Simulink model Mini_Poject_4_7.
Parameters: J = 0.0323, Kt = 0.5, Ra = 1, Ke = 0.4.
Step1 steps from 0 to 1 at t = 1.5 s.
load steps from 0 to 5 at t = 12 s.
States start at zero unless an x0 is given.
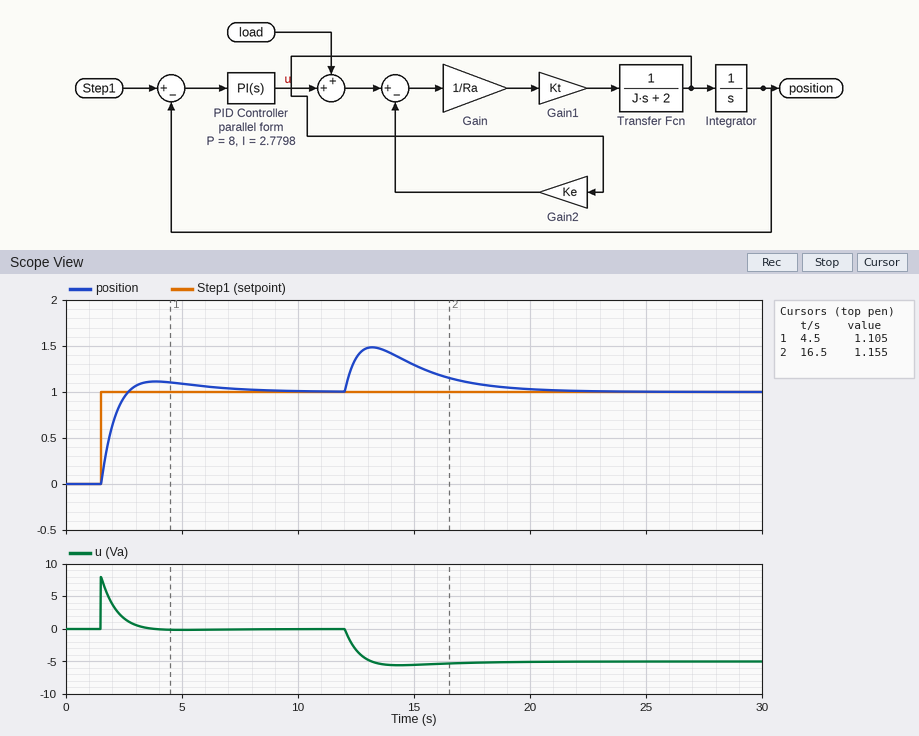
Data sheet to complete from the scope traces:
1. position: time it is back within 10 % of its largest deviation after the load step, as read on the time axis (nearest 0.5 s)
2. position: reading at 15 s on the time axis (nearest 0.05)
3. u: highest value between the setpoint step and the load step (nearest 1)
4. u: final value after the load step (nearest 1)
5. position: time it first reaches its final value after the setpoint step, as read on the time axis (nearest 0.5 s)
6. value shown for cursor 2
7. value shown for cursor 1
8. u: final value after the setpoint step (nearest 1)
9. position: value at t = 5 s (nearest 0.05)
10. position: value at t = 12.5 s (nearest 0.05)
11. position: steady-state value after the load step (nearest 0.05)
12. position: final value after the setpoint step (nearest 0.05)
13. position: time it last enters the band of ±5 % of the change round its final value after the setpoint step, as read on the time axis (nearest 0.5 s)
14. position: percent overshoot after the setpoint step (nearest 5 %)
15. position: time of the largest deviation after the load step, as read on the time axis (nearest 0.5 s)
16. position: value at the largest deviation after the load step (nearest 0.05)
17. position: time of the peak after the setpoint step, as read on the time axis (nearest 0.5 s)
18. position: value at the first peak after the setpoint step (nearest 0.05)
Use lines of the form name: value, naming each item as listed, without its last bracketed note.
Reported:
position: time it is back within 10 % of its largest deviation after the load step, as read on the time axis: 19.0 s
position: reading at 15 s on the time axis: 1.30
u: highest value between the setpoint step and the load step: 8
u: final value after the load step: -5
position: time it first reaches its final value after the setpoint step, as read on the time axis: 2.5 s
value shown for cursor 2: 1.155
value shown for cursor 1: 1.105
u: final value after the setpoint step: 0
position: value at t = 5 s: 1.10
position: value at t = 12.5 s: 1.35
position: steady-state value after the load step: 1.00
position: final value after the setpoint step: 1.00
position: time it last enters the band of ±5 % of the change round its final value after the setpoint step, as read on the time axis: 6.5 s
position: percent overshoot after the setpoint step: 10 %
position: time of the largest deviation after the load step, as read on the time axis: 13.0 s
position: value at the largest deviation after the load step: 1.50
position: time of the peak after the setpoint step, as read on the time axis: 4.0 s
position: value at the first peak after the setpoint step: 1.10
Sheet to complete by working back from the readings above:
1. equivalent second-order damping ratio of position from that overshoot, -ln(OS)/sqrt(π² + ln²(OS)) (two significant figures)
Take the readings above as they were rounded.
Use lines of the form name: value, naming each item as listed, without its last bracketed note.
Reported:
equivalent second-order damping ratio of position from that overshoot, -ln(OS)/sqrt(π² + ln²(OS)): 0.59
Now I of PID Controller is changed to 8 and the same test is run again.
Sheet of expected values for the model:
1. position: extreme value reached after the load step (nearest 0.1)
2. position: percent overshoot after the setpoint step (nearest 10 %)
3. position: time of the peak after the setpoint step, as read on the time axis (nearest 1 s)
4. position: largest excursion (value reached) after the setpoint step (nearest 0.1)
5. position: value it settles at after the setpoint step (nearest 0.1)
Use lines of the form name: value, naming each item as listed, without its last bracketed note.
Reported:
position: extreme value reached after the load step: 1.4
position: percent overshoot after the setpoint step: 20 %
position: time of the peak after the setpoint step, as read on the time axis: 3 s
position: largest excursion (value reached) after the setpoint step: 1.2
position: value it settles at after the setpoint step: 1.0
